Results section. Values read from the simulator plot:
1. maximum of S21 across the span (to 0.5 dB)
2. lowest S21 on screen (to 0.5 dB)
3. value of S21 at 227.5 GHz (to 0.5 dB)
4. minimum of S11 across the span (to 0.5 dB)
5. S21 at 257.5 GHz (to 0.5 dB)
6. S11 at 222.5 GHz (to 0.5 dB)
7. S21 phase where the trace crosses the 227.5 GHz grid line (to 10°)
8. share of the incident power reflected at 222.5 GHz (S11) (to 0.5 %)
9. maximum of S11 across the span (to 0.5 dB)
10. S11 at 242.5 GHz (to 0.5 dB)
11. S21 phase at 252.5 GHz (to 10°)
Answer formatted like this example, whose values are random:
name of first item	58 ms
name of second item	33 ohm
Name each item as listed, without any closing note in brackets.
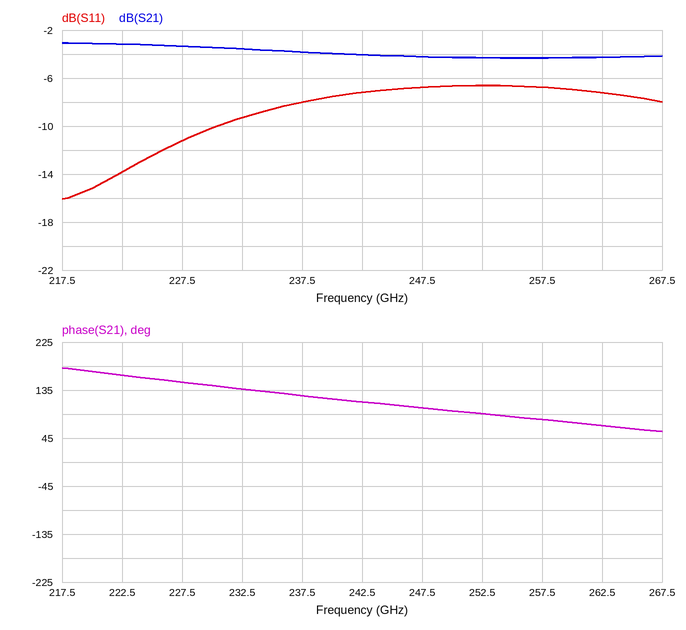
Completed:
maximum of S21 across the span	-3.0 dB
lowest S21 on screen	-4.5 dB
value of S21 at 227.5 GHz	-3.5 dB
minimum of S11 across the span	-16.0 dB
S21 at 257.5 GHz	-4.5 dB
S11 at 222.5 GHz	-14.0 dB
S21 phase where the trace crosses the 227.5 GHz grid line	150°
share of the incident power reflected at 222.5 GHz (S11)	4.0 %
maximum of S11 across the span	-6.5 dB
S11 at 242.5 GHz	-7.0 dB
S21 phase at 252.5 GHz	90°
